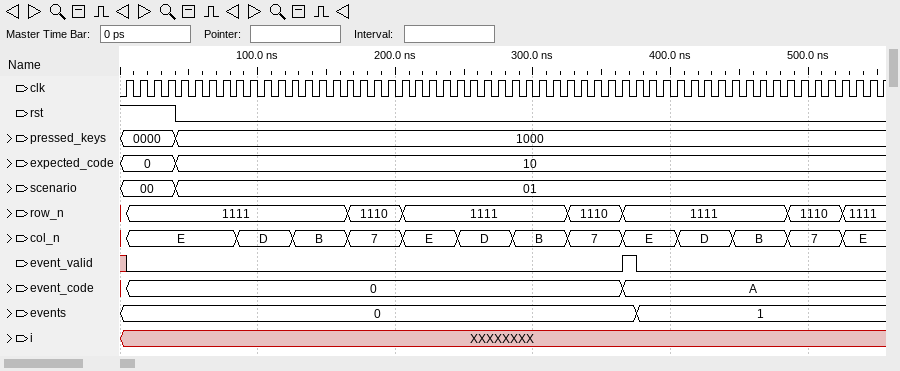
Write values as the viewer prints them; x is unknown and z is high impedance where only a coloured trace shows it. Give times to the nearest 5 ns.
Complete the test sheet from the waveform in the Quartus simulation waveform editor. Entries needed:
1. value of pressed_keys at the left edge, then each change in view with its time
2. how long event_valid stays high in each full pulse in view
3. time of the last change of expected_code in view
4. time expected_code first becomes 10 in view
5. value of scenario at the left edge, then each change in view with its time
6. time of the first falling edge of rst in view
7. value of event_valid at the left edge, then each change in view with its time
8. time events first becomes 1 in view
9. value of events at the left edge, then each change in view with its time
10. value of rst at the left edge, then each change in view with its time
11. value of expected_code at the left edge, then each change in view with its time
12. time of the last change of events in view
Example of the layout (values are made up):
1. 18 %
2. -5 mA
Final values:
1. 0000, 1000 at 40 ns
2. 10 ns
3. 40 ns
4. 40 ns
5. 00, 01 at 40 ns
6. 40 ns
7. x, 0 at 5 ns, 1 at 365 ns, 0 at 375 ns
8. 375 ns
9. 0, 1 at 375 ns
10. 1, 0 at 40 ns
11. 0, 10 at 40 ns
12. 375 ns
